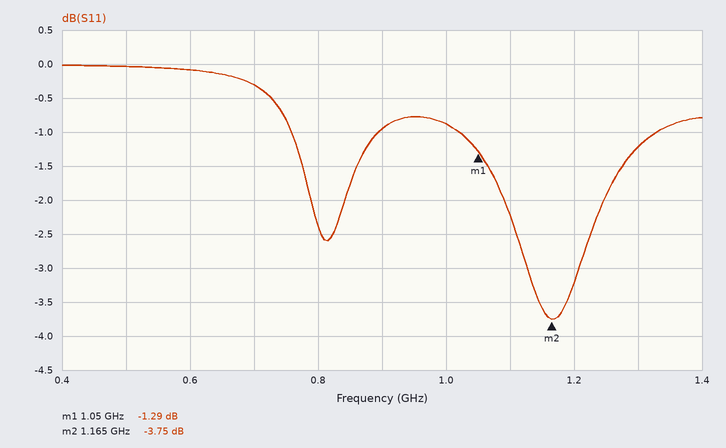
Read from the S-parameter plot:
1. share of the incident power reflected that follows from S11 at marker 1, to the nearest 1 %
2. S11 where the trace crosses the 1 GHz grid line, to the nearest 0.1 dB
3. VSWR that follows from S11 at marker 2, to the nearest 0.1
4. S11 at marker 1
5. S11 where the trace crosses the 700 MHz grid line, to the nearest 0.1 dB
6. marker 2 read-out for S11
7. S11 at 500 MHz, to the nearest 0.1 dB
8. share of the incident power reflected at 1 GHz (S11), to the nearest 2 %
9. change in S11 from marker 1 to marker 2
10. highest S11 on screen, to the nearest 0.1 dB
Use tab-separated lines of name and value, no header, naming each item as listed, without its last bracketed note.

share of the incident power reflected that follows from S11 at marker 1, to the nearest 1 %	74 %
S11 where the trace crosses the 1 GHz grid line, to the nearest 0.1 dB	-0.9 dB
VSWR that follows from S11 at marker 2, to the nearest 0.1	4.7
S11 at marker 1	-1.29 dB
S11 where the trace crosses the 700 MHz grid line, to the nearest 0.1 dB	-0.3 dB
marker 2 read-out for S11	-3.75 dB
S11 at 500 MHz, to the nearest 0.1 dB	0.0 dB
share of the incident power reflected at 1 GHz (S11), to the nearest 2 %	82 %
change in S11 from marker 1 to marker 2	-2.46 dB
highest S11 on screen, to the nearest 0.1 dB	0.0 dB
